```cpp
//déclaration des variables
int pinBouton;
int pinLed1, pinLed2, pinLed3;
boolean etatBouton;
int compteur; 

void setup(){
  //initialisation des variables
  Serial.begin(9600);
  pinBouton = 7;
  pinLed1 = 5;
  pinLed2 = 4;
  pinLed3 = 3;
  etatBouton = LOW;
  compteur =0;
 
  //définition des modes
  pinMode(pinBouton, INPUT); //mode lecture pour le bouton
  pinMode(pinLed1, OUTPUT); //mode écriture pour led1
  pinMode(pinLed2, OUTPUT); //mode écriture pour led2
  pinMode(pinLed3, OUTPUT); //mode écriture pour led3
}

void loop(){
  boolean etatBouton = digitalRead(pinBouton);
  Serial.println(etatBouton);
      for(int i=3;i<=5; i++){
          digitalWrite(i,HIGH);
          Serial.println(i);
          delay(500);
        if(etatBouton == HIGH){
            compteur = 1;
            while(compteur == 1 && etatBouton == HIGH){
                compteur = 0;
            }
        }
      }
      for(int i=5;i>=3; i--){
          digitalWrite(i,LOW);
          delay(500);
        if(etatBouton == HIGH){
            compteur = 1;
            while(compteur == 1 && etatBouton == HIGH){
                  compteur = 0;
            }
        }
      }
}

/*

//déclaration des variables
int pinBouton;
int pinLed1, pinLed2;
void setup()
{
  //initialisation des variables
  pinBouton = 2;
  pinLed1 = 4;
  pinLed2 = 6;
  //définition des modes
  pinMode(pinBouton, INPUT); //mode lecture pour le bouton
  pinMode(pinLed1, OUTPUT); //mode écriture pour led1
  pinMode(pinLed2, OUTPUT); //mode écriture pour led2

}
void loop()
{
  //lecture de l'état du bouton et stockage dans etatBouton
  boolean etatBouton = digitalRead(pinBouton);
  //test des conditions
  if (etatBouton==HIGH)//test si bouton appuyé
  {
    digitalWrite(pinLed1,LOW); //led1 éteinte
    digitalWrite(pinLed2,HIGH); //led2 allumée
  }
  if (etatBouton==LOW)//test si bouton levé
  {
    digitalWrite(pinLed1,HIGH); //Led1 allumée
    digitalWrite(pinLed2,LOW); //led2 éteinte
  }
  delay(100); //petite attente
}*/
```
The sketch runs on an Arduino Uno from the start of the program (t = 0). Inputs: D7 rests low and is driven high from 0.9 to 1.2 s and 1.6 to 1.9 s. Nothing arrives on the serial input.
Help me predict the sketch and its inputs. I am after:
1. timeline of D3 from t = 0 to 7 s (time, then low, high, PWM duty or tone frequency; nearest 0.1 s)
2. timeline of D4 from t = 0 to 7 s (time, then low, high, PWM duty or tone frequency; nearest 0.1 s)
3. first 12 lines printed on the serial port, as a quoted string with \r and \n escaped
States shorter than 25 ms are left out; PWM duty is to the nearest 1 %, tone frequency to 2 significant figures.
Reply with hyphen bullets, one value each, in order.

- 0 s high; 2.5 s low; 3 s high; 5.5 s low; 6 s high
- 0 s low; 0.5 s high; 2 s low; 3.5 s high; 5 s low; 6.5 s high
- "0\r\n3\r\n4\r\n5\r\n0\r\n3\r\n4\r\n5\r\n0\r\n3\r\n4\r\n5\r\n"
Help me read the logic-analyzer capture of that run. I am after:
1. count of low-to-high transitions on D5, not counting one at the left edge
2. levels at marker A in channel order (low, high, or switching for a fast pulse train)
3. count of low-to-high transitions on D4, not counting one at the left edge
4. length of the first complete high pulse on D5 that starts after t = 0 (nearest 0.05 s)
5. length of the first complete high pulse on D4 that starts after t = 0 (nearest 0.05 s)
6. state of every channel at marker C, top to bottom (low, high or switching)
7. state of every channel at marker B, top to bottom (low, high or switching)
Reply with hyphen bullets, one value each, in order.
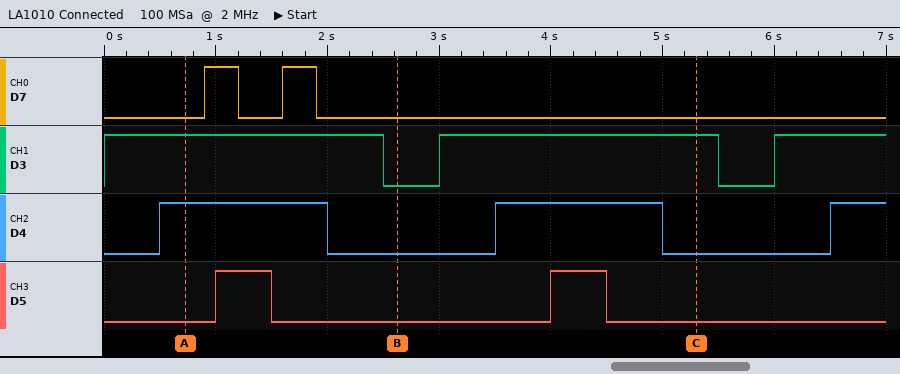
- 2
- D7 low, D3 high, D4 high, D5 low
- 3
- 0.50 s
- 1.50 s
- D7 low, D3 high, D4 low, D5 low
- D7 low, D3 low, D4 low, D5 low
